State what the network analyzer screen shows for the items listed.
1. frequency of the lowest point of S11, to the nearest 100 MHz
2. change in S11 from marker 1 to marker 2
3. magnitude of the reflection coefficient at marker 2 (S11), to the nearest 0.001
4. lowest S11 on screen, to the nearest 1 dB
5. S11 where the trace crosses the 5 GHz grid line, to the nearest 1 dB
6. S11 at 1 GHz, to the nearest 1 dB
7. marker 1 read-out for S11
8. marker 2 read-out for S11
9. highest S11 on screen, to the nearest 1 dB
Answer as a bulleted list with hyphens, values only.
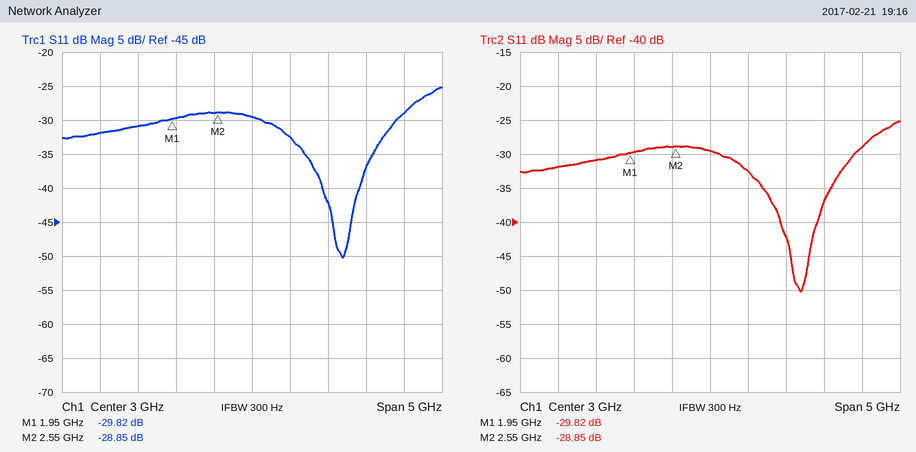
- 4.2 GHz
- 0.97 dB
- 0.036
- -50 dB
- -29 dB
- -32 dB
- -29.82 dB
- -28.85 dB
- -25 dB
